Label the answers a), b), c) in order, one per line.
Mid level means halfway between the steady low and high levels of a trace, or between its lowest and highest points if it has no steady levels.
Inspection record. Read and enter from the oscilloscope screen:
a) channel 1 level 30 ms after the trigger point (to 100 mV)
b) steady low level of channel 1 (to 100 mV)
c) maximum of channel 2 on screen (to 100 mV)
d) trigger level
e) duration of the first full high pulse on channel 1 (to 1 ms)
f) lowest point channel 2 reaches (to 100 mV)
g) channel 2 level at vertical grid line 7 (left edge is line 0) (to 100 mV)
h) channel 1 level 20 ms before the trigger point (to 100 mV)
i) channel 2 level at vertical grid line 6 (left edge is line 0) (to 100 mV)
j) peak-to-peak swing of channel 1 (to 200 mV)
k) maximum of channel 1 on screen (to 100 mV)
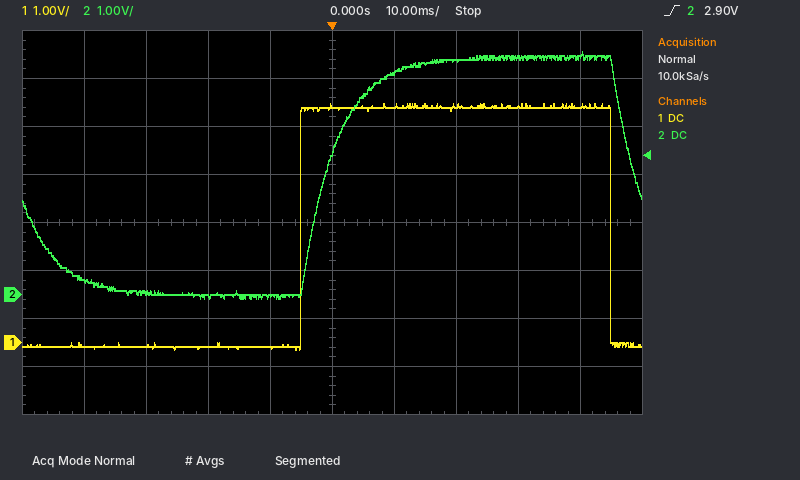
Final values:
a) 4.9 V
b) -100 mV
c) 5.1 V
d) 2.90 V
e) 50 ms
f) -100 mV
g) 4.9 V
h) -100 mV
i) 4.6 V
j) 5.2 V
k) 5.0 V
